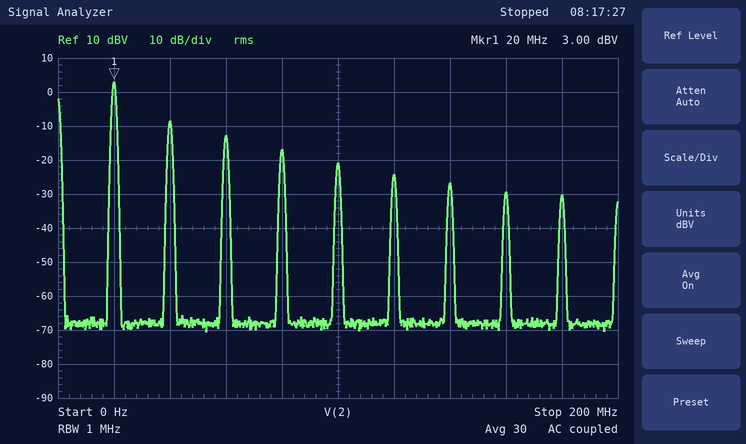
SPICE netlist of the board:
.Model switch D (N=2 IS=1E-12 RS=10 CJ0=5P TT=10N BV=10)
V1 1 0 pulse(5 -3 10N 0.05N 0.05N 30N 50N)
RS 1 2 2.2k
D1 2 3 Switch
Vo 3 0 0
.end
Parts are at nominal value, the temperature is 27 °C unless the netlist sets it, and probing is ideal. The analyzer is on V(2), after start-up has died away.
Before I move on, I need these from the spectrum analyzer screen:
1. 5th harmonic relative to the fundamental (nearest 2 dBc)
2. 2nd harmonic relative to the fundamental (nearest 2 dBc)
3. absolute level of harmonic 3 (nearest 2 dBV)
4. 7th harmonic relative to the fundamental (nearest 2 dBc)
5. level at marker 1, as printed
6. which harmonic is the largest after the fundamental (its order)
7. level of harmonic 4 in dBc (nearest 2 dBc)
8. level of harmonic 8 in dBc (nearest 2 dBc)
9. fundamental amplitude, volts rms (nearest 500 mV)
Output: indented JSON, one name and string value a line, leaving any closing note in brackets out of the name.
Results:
{
  "5th harmonic relative to the fundamental": "-24 dBc",
  "2nd harmonic relative to the fundamental": "-12 dBc",
  "absolute level of harmonic 3": "-12 dBV",
  "7th harmonic relative to the fundamental": "-30 dBc",
  "level at marker 1, as printed": "3.00 dBV",
  "which harmonic is the largest after the fundamental": "2",
  "level of harmonic 4 in dBc": "-20 dBc",
  "level of harmonic 8 in dBc": "-32 dBc",
  "fundamental amplitude, volts rms": "1.5 V"
}
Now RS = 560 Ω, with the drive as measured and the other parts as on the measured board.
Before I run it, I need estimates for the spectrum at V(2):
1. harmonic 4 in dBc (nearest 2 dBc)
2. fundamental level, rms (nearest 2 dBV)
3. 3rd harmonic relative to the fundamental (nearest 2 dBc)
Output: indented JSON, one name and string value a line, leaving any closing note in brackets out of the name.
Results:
{
  "harmonic 4 in dBc": "-18 dBc",
  "fundamental level, rms": "6 dBV",
  "3rd harmonic relative to the fundamental": "-12 dBc"
}
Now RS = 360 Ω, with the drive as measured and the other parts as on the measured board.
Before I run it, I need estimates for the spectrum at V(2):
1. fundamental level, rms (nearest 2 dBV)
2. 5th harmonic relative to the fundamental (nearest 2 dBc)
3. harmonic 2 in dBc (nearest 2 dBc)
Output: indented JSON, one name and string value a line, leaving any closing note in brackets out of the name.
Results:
{
  "fundamental level, rms": "6 dBV",
  "5th harmonic relative to the fundamental": "-18 dBc",
  "harmonic 2 in dBc": "-20 dBc"
}
